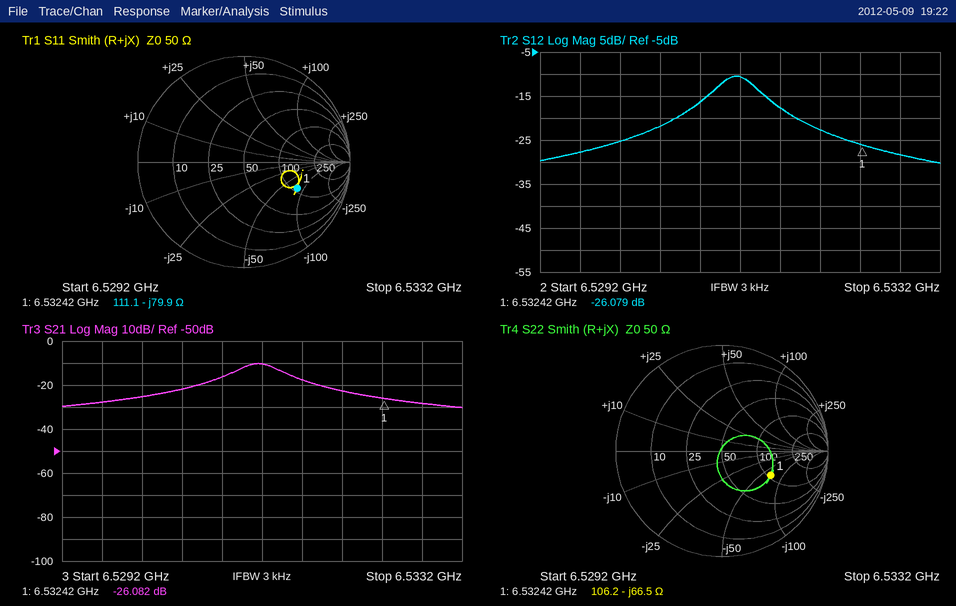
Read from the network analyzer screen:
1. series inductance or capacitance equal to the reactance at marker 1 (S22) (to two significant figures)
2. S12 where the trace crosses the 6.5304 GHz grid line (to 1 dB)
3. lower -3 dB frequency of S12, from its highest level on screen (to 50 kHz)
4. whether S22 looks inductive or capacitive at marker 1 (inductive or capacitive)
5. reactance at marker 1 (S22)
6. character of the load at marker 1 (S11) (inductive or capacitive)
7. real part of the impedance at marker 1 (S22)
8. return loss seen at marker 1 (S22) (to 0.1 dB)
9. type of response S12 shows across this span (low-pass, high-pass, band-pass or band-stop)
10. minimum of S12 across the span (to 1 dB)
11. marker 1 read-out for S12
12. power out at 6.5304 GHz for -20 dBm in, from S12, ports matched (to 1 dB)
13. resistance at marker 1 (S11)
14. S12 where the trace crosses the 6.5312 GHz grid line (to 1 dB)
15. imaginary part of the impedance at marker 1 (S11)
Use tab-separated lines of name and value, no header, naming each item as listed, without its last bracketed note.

series inductance or capacitance equal to the reactance at marker 1 (S22)	370 fF
S12 where the trace crosses the 6.5304 GHz grid line	-22 dB
lower -3 dB frequency of S12, from its highest level on screen	6.53095 GHz
whether S22 looks inductive or capacitive at marker 1	capacitive
reactance at marker 1	-66.5 Ω
character of the load at marker 1 (S11)	capacitive
real part of the impedance at marker 1	106.2 Ω
return loss seen at marker 1 (S22)	5.8 dB
type of response S12 shows across this span	band-pass
minimum of S12 across the span	-30 dB
marker 1 read-out for S12	-26.079 dB
power out at 6.5304 GHz for -20 dBm in, from S12, ports matched	-42 dBm
resistance at marker 1	111.1 Ω
S12 where the trace crosses the 6.5312 GHz grid line	-11 dB
imaginary part of the impedance at marker 1	-79.9 Ω
